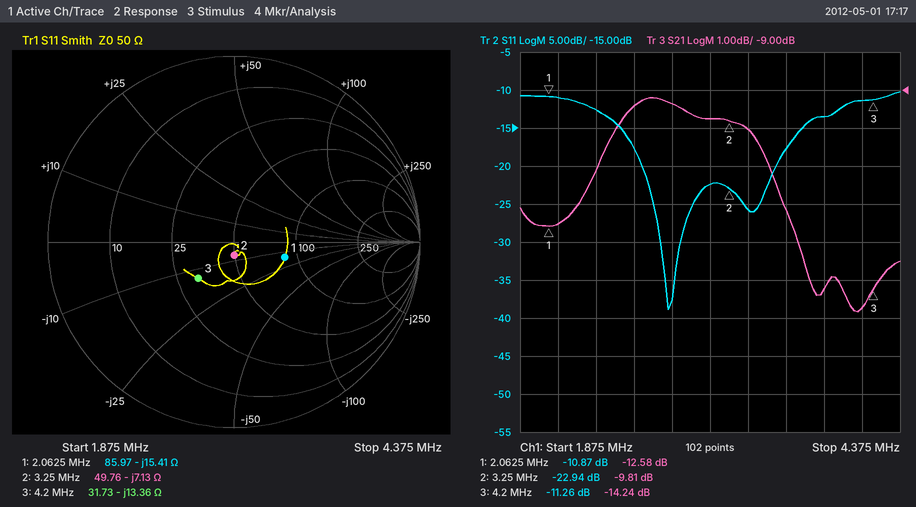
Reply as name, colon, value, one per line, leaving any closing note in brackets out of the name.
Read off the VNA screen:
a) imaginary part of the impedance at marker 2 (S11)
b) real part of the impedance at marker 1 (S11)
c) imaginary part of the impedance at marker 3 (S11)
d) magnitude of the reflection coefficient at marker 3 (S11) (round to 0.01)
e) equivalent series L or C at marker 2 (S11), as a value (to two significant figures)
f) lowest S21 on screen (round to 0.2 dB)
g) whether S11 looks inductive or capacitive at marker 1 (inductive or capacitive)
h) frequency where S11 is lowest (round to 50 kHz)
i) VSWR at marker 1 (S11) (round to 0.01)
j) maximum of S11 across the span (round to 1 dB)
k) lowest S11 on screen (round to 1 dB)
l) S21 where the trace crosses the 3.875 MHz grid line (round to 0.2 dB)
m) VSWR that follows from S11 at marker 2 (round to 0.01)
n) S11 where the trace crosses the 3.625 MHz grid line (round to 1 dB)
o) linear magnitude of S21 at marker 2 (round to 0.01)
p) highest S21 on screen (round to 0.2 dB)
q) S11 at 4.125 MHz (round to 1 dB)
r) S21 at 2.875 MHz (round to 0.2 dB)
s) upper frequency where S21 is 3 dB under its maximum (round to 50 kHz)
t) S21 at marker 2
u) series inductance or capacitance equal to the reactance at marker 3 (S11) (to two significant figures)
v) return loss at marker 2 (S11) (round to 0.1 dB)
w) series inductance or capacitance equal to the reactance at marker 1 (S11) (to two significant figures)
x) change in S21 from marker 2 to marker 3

imaginary part of the impedance at marker 2: -7.13 Ω
real part of the impedance at marker 1: 85.97 Ω
imaginary part of the impedance at marker 3: -13.36 Ω
magnitude of the reflection coefficient at marker 3 (S11): 0.27
equivalent series L or C at marker 2 (S11), as a value: 6.9 nF
lowest S21 on screen: -14.8 dB
whether S11 looks inductive or capacitive at marker 1: capacitive
frequency where S11 is lowest: 2.85 MHz
VSWR at marker 1 (S11): 1.80
maximum of S11 across the span: -10 dB
lowest S11 on screen: -39 dB
S21 where the trace crosses the 3.875 MHz grid line: -14.2 dB
VSWR that follows from S11 at marker 2: 1.15
S11 where the trace crosses the 3.625 MHz grid line: -18 dB
linear magnitude of S21 at marker 2: 0.32
highest S21 on screen: -9.2 dB
S11 at 4.125 MHz: -11 dB
S21 at 2.875 MHz: -9.4 dB
upper frequency where S21 is 3 dB under its maximum: 3.65 MHz
S21 at marker 2: -9.81 dB
series inductance or capacitance equal to the reactance at marker 3 (S11): 2.8 nF
return loss at marker 2 (S11): 22.9 dB
series inductance or capacitance equal to the reactance at marker 1 (S11): 5.0 nF
change in S21 from marker 2 to marker 3: -4.43 dB
